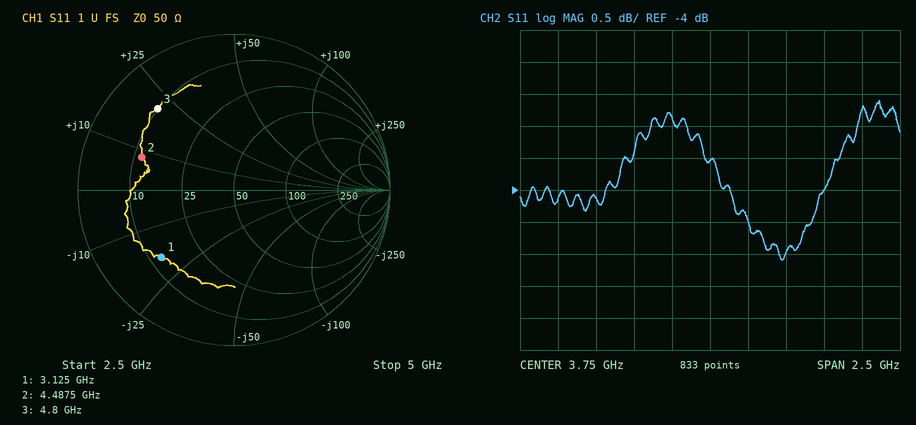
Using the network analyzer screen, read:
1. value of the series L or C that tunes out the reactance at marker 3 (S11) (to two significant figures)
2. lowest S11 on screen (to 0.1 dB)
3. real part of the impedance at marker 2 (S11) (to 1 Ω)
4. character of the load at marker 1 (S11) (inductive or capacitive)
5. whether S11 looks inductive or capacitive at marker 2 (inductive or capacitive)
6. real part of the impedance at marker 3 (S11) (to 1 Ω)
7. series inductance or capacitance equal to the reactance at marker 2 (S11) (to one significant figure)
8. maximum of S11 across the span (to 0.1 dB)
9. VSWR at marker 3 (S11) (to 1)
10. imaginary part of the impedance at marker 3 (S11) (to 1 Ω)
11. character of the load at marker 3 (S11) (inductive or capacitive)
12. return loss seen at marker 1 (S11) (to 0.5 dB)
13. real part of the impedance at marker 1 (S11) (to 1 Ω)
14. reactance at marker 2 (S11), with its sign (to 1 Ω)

1.6 pF
-5.1 dB
12 Ω
capacitive
inductive
10 Ω
300 pH
-2.6 dB
6
+21 Ω
inductive
4.0 dB
13 Ω
+8 Ω
